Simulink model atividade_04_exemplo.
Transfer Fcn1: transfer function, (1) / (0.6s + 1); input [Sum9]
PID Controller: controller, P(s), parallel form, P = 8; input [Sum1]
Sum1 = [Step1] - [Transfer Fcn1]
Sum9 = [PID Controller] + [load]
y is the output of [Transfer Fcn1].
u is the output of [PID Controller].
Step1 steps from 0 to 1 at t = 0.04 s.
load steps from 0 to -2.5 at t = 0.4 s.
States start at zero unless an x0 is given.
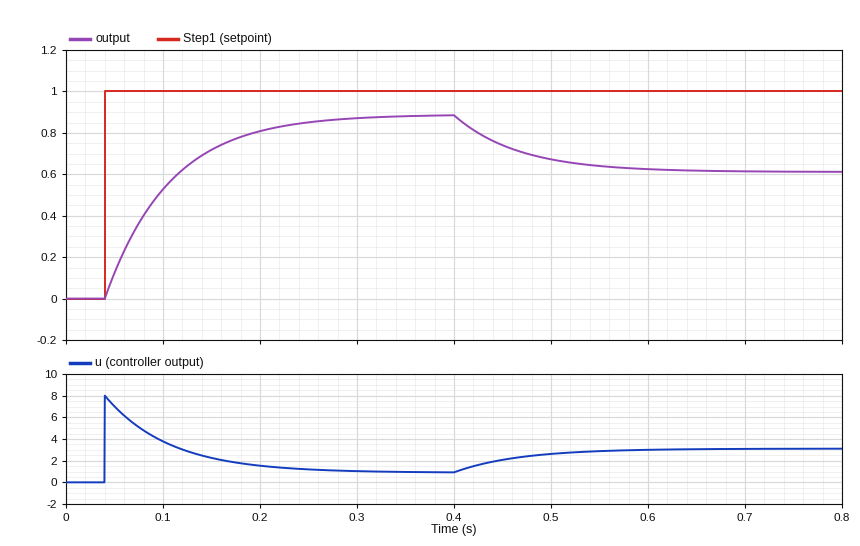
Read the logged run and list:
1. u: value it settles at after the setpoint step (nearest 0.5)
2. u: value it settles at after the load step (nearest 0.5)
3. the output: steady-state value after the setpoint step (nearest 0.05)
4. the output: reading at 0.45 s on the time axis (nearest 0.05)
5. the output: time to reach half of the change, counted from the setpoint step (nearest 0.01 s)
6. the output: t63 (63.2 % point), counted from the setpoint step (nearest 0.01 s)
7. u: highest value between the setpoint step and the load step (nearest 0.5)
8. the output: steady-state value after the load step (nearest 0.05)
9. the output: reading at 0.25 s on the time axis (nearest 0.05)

1.0
3.0
0.90
0.75
0.05 s
0.07 s
8.0
0.60
0.85
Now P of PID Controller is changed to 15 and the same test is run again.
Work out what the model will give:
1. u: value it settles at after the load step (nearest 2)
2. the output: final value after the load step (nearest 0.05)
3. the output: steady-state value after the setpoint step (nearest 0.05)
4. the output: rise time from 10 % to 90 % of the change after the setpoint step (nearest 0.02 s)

4
0.80
0.95
0.08 s
